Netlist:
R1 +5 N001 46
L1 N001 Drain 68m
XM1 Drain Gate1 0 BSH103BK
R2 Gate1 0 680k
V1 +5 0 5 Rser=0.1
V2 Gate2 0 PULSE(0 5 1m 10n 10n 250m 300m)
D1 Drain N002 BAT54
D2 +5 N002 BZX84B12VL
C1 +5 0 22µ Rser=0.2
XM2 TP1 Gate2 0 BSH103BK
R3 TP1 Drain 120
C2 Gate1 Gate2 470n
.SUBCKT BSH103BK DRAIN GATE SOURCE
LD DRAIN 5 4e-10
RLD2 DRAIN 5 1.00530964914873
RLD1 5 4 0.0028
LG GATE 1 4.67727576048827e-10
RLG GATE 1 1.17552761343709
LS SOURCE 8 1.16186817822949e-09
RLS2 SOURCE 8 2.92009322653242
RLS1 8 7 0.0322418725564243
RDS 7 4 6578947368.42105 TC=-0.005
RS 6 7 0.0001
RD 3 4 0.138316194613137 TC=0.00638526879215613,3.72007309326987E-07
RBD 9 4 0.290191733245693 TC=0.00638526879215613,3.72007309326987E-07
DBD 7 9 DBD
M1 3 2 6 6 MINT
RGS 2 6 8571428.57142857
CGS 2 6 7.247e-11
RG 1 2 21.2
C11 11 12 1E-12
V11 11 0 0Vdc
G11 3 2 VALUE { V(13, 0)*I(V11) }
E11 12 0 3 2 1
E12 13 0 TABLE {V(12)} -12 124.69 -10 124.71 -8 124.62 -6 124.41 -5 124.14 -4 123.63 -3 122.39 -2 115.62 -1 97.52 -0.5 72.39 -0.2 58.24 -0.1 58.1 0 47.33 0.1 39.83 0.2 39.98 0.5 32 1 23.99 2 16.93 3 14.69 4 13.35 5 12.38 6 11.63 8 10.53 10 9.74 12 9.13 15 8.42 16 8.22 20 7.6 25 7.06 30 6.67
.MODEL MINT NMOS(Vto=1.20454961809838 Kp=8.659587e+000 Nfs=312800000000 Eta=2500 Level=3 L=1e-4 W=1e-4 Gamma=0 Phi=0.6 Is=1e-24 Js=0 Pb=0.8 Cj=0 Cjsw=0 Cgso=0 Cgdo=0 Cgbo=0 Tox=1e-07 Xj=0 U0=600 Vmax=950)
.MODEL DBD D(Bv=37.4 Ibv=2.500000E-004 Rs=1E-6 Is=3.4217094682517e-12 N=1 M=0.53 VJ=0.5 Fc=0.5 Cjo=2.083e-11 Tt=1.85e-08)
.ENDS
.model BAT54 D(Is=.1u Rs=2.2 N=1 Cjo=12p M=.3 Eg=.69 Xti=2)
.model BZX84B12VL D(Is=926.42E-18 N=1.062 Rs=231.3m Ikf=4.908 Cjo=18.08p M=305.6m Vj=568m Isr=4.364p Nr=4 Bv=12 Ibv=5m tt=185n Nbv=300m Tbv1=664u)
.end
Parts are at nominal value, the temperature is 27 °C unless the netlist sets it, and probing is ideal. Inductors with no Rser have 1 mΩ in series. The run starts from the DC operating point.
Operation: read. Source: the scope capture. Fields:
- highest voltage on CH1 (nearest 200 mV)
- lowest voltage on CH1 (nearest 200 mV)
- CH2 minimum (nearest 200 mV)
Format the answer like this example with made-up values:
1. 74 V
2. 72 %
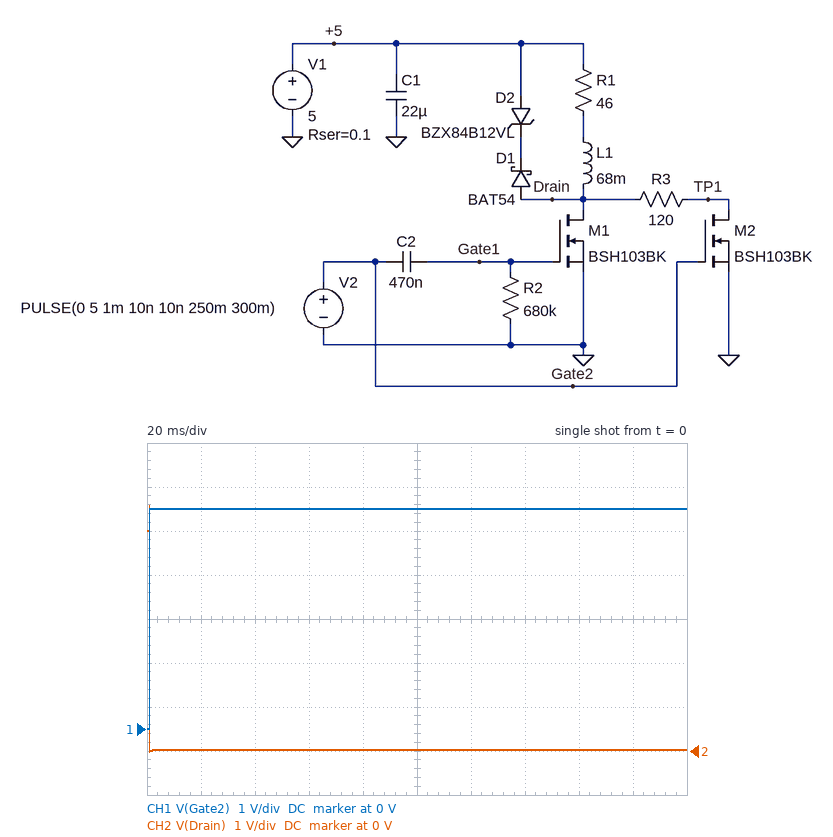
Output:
1. 5.0 V
2. 0 V
3. 0 V
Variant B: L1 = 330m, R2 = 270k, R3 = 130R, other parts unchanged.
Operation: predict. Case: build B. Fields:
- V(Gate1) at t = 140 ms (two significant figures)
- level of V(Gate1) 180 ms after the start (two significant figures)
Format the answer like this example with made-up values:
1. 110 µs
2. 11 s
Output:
1. 1.6 V
2. 1.2 V
